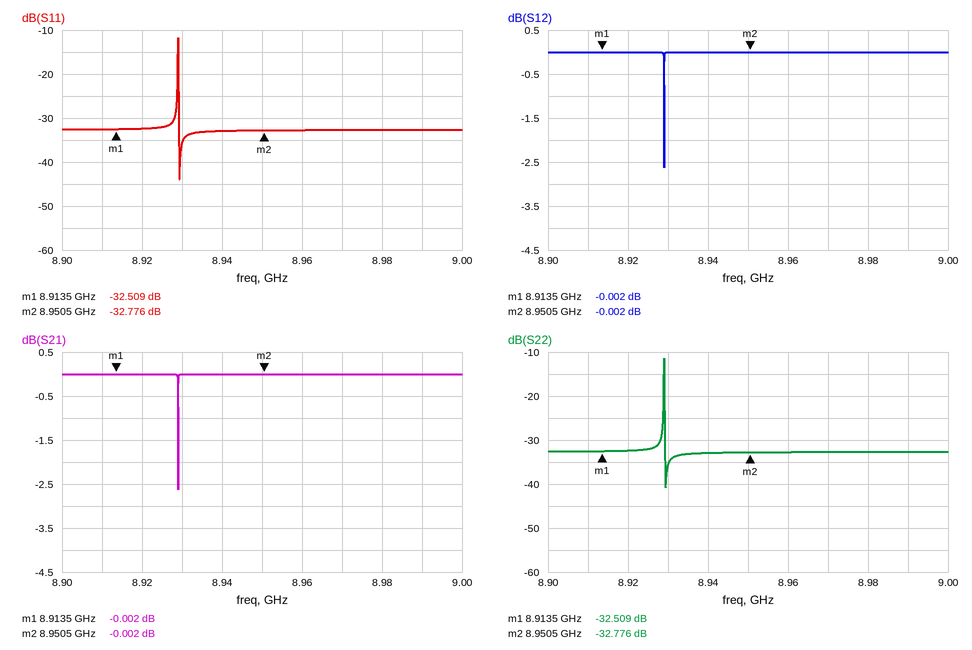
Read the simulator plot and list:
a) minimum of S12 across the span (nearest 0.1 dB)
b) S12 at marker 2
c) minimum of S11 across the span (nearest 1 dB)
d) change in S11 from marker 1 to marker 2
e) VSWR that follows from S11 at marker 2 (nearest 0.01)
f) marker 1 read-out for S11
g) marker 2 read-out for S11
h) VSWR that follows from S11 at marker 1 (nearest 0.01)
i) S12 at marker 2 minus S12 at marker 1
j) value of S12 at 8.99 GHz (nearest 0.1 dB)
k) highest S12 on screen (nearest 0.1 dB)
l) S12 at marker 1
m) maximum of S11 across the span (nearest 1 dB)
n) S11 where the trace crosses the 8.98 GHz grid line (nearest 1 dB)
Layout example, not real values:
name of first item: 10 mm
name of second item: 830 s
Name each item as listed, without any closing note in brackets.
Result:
minimum of S12 across the span: -2.6 dB
S12 at marker 2: -0.002 dB
minimum of S11 across the span: -44 dB
change in S11 from marker 1 to marker 2: -0.267 dB
VSWR that follows from S11 at marker 2: 1.05
marker 1 read-out for S11: -32.509 dB
marker 2 read-out for S11: -32.776 dB
VSWR that follows from S11 at marker 1: 1.05
S12 at marker 2 minus S12 at marker 1: 0.000 dB
value of S12 at 8.99 GHz: 0.0 dB
highest S12 on screen: 0.0 dB
S12 at marker 1: -0.002 dB
maximum of S11 across the span: -12 dB
S11 where the trace crosses the 8.98 GHz grid line: -33 dB
